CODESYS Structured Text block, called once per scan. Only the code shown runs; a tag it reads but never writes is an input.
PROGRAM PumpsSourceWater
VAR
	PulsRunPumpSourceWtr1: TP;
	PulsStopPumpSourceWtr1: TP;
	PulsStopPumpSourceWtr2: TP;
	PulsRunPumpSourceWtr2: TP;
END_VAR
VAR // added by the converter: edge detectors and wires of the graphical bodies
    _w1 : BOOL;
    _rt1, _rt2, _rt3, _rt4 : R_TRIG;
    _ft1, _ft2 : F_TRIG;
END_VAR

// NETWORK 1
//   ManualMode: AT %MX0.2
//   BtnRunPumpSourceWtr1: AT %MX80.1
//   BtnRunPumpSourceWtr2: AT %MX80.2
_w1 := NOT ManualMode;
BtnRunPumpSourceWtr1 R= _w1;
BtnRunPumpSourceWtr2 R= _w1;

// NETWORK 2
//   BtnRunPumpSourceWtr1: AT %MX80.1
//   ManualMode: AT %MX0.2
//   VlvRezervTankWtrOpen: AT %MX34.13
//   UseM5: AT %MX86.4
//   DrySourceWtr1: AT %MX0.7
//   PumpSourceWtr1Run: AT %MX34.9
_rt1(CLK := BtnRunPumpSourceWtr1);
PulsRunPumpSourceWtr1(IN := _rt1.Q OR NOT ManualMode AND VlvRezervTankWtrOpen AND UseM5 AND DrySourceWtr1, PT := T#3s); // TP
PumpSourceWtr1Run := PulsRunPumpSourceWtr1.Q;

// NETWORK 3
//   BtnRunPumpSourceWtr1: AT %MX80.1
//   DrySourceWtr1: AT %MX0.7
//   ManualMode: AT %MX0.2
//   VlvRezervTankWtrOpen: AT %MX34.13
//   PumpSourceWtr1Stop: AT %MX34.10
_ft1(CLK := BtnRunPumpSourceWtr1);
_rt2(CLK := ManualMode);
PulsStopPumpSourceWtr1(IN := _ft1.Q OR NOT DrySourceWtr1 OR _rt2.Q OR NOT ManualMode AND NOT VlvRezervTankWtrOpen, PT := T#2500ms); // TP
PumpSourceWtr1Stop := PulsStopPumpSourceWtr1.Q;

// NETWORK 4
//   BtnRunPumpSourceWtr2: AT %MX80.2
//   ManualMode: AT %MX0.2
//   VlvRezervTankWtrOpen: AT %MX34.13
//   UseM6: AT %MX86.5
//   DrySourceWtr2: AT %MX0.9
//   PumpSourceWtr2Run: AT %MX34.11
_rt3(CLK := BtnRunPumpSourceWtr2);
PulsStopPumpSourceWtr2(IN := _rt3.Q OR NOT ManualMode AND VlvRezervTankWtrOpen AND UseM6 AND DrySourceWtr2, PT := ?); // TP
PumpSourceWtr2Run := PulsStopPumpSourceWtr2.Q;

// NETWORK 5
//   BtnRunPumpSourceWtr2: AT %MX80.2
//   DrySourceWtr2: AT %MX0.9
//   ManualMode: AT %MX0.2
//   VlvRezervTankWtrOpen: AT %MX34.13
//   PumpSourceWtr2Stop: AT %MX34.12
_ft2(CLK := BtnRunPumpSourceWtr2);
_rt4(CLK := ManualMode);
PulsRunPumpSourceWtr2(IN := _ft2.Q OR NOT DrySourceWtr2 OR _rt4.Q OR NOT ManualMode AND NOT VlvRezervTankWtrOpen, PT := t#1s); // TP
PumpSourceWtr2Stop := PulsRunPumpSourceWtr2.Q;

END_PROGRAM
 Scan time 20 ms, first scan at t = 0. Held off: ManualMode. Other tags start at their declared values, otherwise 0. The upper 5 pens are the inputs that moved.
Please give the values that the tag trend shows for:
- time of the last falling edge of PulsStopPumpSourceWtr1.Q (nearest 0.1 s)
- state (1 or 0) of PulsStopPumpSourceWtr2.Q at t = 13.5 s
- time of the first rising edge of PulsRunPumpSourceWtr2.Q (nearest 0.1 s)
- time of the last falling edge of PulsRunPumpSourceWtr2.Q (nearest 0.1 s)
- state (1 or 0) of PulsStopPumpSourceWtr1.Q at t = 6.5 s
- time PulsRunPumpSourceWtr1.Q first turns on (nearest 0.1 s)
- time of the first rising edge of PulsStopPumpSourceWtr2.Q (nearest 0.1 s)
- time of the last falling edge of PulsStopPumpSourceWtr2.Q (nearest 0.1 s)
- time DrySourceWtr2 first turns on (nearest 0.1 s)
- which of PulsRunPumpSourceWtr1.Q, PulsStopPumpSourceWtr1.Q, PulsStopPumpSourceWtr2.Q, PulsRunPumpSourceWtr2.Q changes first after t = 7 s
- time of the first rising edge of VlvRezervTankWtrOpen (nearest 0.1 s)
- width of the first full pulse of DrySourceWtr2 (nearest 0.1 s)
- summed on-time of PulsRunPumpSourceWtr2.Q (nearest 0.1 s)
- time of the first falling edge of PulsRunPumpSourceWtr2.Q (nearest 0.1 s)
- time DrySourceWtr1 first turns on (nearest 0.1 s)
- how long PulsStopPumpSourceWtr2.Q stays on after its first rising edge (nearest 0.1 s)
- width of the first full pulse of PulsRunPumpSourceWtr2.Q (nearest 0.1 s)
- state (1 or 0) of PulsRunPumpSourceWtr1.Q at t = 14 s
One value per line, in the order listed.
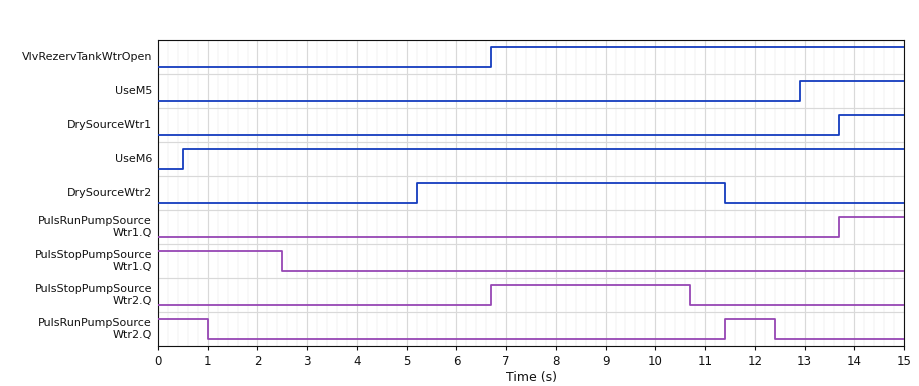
2.5 s
0
11.4 s
12.4 s
0
13.7 s
6.7 s
10.7 s
5.2 s
PulsStopPumpSourceWtr2.Q
6.7 s
6.2 s
2.0 s
1.0 s
13.7 s
4.0 s
1.0 s
1
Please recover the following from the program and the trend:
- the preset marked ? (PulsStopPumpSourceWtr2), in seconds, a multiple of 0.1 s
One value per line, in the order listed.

4.0 s
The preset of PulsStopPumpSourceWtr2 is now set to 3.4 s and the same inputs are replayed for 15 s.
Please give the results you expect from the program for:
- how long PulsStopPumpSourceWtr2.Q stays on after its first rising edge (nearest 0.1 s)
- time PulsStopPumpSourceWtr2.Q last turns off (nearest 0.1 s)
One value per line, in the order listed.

3.4 s
10.1 s
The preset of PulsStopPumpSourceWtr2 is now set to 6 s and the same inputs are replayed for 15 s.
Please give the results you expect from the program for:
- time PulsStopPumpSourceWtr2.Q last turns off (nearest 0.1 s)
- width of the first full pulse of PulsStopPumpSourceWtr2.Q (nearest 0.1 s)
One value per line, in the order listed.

12.7 s
6.0 s
